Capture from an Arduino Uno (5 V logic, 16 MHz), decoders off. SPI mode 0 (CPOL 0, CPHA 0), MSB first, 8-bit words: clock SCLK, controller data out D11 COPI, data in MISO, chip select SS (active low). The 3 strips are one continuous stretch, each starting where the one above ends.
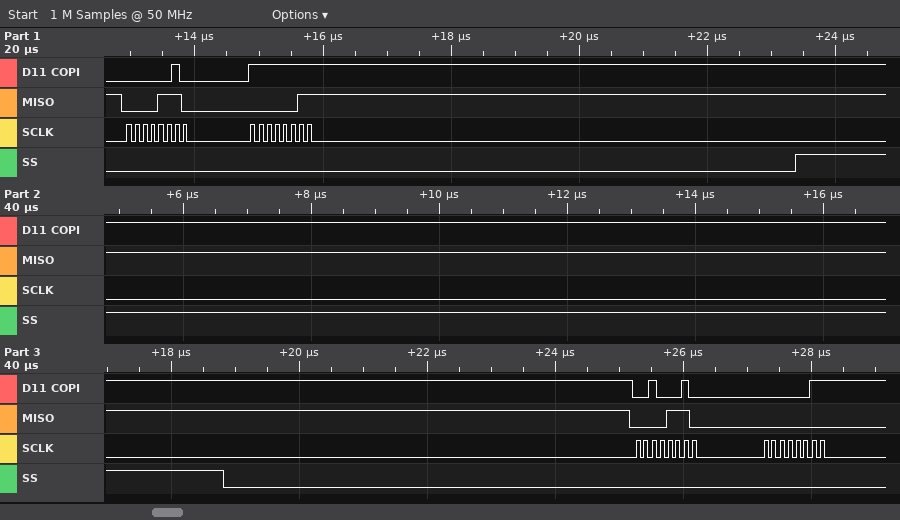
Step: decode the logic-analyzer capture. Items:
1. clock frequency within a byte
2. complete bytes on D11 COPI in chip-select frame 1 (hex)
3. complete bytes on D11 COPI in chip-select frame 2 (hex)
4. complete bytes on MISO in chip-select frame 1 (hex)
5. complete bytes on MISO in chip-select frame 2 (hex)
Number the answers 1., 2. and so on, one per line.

1. 8 MHz
2. 0x02 0xFF
3. 0x22 0x03
4. 0x0E 0x03
5. 0x0E 0x00
